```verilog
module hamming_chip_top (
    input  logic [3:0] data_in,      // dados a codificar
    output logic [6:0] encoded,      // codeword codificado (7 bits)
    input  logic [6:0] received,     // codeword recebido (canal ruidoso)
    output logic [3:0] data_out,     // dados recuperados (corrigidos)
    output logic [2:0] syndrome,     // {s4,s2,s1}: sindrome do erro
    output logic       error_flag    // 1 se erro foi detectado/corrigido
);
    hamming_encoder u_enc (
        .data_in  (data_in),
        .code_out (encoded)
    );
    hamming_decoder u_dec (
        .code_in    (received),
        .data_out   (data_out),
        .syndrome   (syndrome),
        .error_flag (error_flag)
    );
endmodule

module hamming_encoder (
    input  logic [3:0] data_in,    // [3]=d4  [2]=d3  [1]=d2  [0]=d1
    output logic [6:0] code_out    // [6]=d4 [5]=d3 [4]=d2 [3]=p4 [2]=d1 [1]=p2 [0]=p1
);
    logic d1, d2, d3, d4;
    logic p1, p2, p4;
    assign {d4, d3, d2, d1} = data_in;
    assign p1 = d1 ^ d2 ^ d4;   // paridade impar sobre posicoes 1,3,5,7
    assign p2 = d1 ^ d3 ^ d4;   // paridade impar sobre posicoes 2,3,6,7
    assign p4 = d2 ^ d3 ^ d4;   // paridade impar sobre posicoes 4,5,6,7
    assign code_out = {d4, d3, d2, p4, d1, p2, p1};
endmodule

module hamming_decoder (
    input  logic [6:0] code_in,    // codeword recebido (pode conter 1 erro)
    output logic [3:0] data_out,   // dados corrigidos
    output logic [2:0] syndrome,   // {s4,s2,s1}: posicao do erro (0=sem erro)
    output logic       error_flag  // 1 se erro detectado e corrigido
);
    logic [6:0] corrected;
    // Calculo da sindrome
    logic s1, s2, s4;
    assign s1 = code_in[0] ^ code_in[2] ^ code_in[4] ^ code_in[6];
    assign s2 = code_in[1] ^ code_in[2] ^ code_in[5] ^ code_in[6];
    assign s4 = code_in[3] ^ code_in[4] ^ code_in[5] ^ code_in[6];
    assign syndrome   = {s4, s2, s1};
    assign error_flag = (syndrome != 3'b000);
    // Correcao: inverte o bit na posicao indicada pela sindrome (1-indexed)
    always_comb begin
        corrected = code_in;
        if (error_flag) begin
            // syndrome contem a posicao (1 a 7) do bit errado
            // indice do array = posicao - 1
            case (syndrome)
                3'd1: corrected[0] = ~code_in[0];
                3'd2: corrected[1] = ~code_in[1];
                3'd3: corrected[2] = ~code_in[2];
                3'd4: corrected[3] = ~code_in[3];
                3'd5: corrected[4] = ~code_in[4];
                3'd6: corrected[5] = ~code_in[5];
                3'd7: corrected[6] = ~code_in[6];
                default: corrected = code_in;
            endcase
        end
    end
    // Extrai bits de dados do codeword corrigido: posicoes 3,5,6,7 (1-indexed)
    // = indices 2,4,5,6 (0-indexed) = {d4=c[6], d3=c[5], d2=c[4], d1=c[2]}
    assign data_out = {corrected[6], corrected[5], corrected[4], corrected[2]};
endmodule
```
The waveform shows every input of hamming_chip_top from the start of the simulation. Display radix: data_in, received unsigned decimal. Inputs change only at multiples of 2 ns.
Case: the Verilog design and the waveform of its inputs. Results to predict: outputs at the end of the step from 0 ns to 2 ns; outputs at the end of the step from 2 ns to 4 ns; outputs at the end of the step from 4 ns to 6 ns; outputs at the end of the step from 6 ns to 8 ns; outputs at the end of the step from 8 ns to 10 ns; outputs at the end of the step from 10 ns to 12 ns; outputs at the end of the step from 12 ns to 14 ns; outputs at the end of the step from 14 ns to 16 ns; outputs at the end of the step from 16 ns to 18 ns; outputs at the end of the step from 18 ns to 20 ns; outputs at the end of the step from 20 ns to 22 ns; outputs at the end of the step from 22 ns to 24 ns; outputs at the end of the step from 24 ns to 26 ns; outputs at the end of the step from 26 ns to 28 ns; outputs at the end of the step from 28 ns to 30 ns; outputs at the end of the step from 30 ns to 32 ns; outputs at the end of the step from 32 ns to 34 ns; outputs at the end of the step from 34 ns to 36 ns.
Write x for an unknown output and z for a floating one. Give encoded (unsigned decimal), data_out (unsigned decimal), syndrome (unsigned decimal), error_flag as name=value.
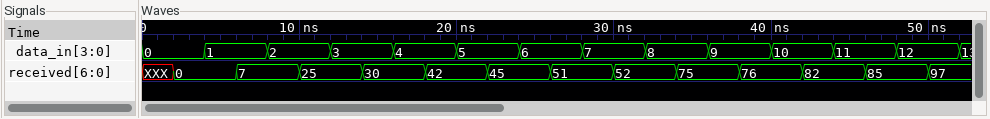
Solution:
encoded=0, data_out=x, syndrome=x, error_flag=x
encoded=0, data_out=0, syndrome=0, error_flag=0
encoded=7, data_out=0, syndrome=0, error_flag=0
encoded=7, data_out=1, syndrome=0, error_flag=0
encoded=25, data_out=1, syndrome=0, error_flag=0
encoded=25, data_out=2, syndrome=0, error_flag=0
encoded=30, data_out=2, syndrome=0, error_flag=0
encoded=30, data_out=3, syndrome=0, error_flag=0
encoded=42, data_out=3, syndrome=0, error_flag=0
encoded=42, data_out=4, syndrome=0, error_flag=0
encoded=45, data_out=4, syndrome=0, error_flag=0
encoded=45, data_out=5, syndrome=0, error_flag=0
encoded=51, data_out=5, syndrome=0, error_flag=0
encoded=51, data_out=6, syndrome=0, error_flag=0
encoded=52, data_out=6, syndrome=0, error_flag=0
encoded=52, data_out=7, syndrome=0, error_flag=0
encoded=75, data_out=7, syndrome=0, error_flag=0
encoded=75, data_out=8, syndrome=0, error_flag=0
